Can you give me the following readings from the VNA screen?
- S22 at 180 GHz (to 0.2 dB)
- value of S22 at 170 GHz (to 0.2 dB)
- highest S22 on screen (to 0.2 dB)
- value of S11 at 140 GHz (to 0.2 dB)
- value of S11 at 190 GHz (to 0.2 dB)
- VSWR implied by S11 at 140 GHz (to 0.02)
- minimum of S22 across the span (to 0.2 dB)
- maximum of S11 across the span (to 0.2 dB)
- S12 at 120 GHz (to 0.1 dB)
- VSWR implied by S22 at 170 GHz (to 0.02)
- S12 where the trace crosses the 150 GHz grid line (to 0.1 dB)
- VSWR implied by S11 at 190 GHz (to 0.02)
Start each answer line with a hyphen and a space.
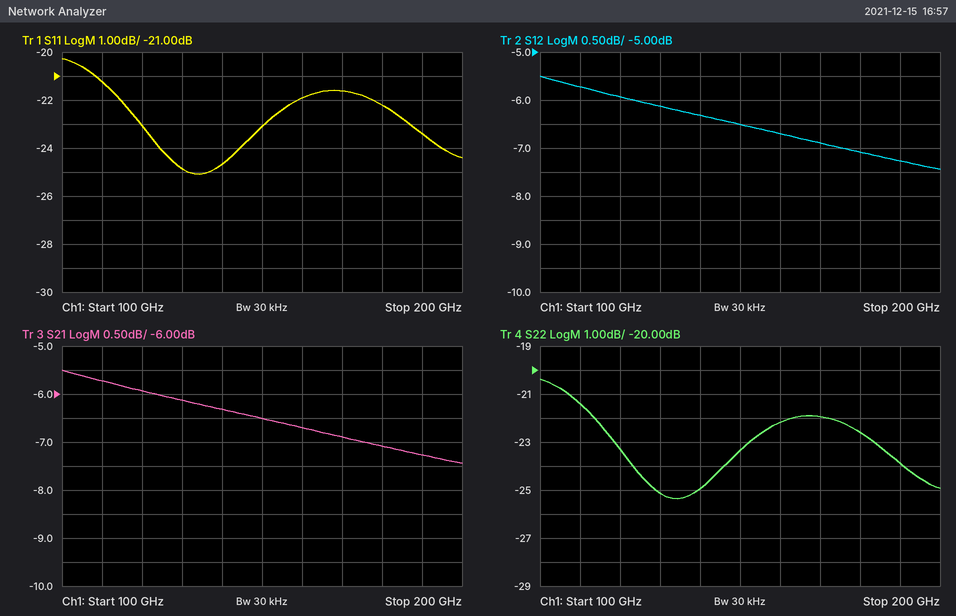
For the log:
- -22.6 dB
- -22.0 dB
- -20.4 dB
- -24.6 dB
- -23.4 dB
- 1.12
- -25.4 dB
- -20.2 dB
- -5.9 dB
- 1.18
- -6.5 dB
- 1.14
